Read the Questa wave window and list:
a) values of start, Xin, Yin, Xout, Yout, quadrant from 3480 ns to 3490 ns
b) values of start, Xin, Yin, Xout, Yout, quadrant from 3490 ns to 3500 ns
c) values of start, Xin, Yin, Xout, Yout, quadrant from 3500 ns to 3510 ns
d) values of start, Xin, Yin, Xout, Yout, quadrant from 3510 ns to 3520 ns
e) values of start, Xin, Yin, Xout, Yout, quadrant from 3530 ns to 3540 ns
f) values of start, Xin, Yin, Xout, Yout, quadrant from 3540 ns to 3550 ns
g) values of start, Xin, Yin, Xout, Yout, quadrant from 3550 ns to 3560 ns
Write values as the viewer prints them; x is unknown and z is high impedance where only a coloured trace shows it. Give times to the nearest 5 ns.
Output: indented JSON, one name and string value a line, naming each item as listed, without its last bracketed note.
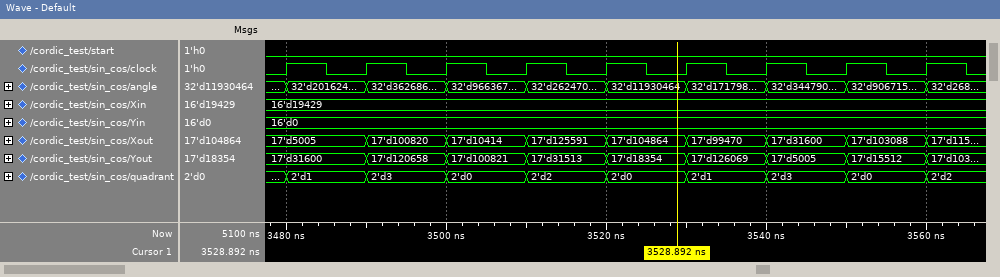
{
  "values of start, Xin, Yin, Xout, Yout, quadrant from 3480 ns to 3490 ns": "start=0, Xin=16'd19429, Yin=16'd0, Xout=17'd5005, Yout=17'd31600, quadrant=2'd1",
  "values of start, Xin, Yin, Xout, Yout, quadrant from 3490 ns to 3500 ns": "start=0, Xin=16'd19429, Yin=16'd0, Xout=17'd100820, Yout=17'd120658, quadrant=2'd3",
  "values of start, Xin, Yin, Xout, Yout, quadrant from 3500 ns to 3510 ns": "start=0, Xin=16'd19429, Yin=16'd0, Xout=17'd10414, Yout=17'd100821, quadrant=2'd0",
  "values of start, Xin, Yin, Xout, Yout, quadrant from 3510 ns to 3520 ns": "start=0, Xin=16'd19429, Yin=16'd0, Xout=17'd125591, Yout=17'd31513, quadrant=2'd2",
  "values of start, Xin, Yin, Xout, Yout, quadrant from 3530 ns to 3540 ns": "start=0, Xin=16'd19429, Yin=16'd0, Xout=17'd99470, Yout=17'd126069, quadrant=2'd1",
  "values of start, Xin, Yin, Xout, Yout, quadrant from 3540 ns to 3550 ns": "start=0, Xin=16'd19429, Yin=16'd0, Xout=17'd31600, Yout=17'd5005, quadrant=2'd3",
  "values of start, Xin, Yin, Xout, Yout, quadrant from 3550 ns to 3560 ns": "start=0, Xin=16'd19429, Yin=16'd0, Xout=17'd103088, Yout=17'd15512, quadrant=2'd0"
}
